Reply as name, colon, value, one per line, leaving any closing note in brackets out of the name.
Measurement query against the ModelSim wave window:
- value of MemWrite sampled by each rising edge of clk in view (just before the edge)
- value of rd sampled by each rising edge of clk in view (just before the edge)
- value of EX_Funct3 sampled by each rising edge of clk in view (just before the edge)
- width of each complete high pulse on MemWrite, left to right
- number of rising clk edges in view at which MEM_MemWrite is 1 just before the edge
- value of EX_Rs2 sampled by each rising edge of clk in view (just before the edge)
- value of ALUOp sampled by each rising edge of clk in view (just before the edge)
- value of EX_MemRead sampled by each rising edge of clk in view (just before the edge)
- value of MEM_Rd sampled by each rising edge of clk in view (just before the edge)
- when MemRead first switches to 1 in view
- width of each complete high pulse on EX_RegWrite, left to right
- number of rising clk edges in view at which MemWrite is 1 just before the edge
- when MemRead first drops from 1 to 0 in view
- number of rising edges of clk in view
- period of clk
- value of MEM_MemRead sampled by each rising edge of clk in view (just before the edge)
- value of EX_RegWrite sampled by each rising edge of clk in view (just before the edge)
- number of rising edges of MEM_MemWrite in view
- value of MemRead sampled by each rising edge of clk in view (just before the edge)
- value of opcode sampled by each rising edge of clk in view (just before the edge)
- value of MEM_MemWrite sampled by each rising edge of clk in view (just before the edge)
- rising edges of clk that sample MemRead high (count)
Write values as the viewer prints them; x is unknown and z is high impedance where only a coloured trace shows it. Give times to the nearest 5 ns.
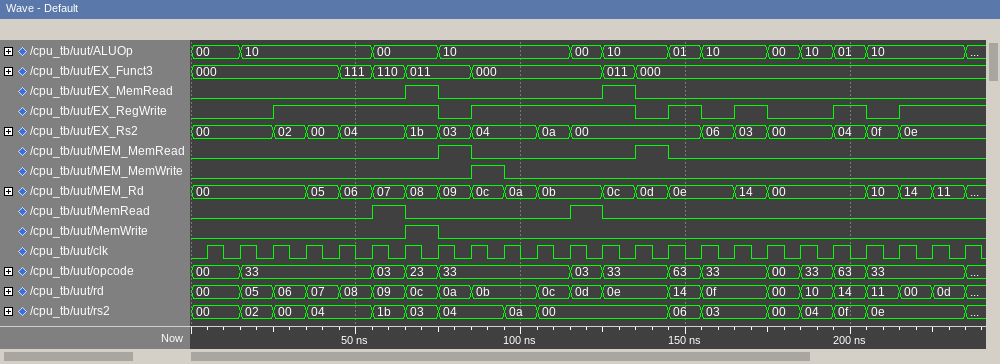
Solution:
value of MemWrite sampled by each rising edge of clk in view: 0 0 0 0 0 0 0 1 0 0 0 0 0 0 0 0 0 0 0 0 0 0 0 0
value of rd sampled by each rising edge of clk in view: 00, 00, 05, 06, 07, 08, 09, 0c, 0a, 0b, 0b, 0c, 0d, 0e, 0e, 14, 0f, 0f, 00, 10, 14, 11, 00, 0d
value of EX_Funct3 sampled by each rising edge of clk in view: 000, 000, 000, 000, 000, 111, 110, 011, 011, 000, 000, 000, 000, 011, 000, 000, 000, 000, 000, 000, 000, 000, 000, 000
width of each complete high pulse on MemWrite, left to right: 10 ns
number of rising clk edges in view at which MEM_MemWrite is 1 just before the edge: 1
value of EX_Rs2 sampled by each rising edge of clk in view: 00, 00, 00, 02, 00, 04, 04, 1b, 03, 04, 04, 0a, 00, 00, 00, 00, 06, 03, 00, 00, 04, 0f, 0e, 0e
value of ALUOp sampled by each rising edge of clk in view: 00, 00, 10, 10, 10, 10, 00, 00, 10, 10, 10, 10, 00, 10, 10, 01, 10, 10, 00, 10, 01, 10, 10, 10
value of EX_MemRead sampled by each rising edge of clk in view: 0 0 0 0 0 0 0 1 0 0 0 0 0 1 0 0 0 0 0 0 0 0 0 0
value of MEM_Rd sampled by each rising edge of clk in view: 00, 00, 00, 00, 05, 06, 07, 08, 09, 0c, 0a, 0b, 0b, 0c, 0d, 0e, 0e, 14, 00, 00, 00, 10, 14, 11
when MemRead first switches to 1 in view: 55 ns
width of each complete high pulse on EX_RegWrite, left to right: 50 ns, 50 ns, 10 ns, 10 ns, 10 ns
number of rising clk edges in view at which MemWrite is 1 just before the edge: 1
when MemRead first drops from 1 to 0 in view: 65 ns
number of rising edges of clk in view: 24
period of clk: 10 ns
value of MEM_MemRead sampled by each rising edge of clk in view: 0 0 0 0 0 0 0 0 1 0 0 0 0 0 1 0 0 0 0 0 0 0 0 0
value of EX_RegWrite sampled by each rising edge of clk in view: 0 0 0 1 1 1 1 1 0 1 1 1 1 1 0 1 0 1 0 0 1 0 1 1
number of rising edges of MEM_MemWrite in view: 1
value of MemRead sampled by each rising edge of clk in view: 0 0 0 0 0 0 1 0 0 0 0 0 1 0 0 0 0 0 0 0 0 0 0 0
value of opcode sampled by each rising edge of clk in view: 00, 00, 33, 33, 33, 33, 03, 23, 33, 33, 33, 33, 03, 33, 33, 63, 33, 33, 00, 33, 63, 33, 33, 33
value of MEM_MemWrite sampled by each rising edge of clk in view: 0 0 0 0 0 0 0 0 0 1 0 0 0 0 0 0 0 0 0 0 0 0 0 0
rising edges of clk that sample MemRead high: 2
